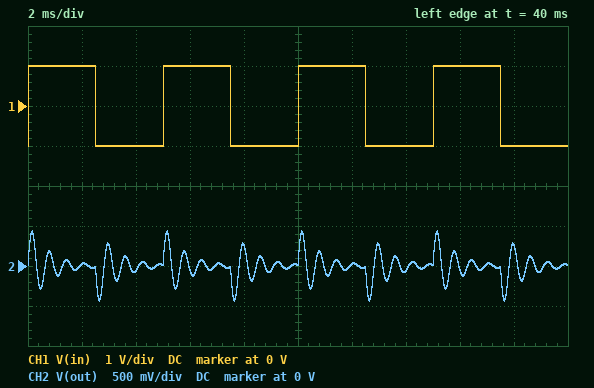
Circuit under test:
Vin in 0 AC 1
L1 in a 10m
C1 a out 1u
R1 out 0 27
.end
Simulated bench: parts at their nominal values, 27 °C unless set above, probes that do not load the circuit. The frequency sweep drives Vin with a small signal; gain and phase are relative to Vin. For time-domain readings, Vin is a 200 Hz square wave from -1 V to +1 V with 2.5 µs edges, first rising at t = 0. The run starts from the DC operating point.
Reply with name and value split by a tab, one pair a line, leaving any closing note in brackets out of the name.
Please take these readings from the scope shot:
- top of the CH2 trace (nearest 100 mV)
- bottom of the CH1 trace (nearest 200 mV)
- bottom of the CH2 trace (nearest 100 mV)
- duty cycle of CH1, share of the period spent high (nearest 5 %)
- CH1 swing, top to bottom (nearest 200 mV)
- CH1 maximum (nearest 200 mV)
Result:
top of the CH2 trace	400 mV
bottom of the CH1 trace	-1.0 V
bottom of the CH2 trace	-400 mV
duty cycle of CH1, share of the period spent high	50 %
CH1 swing, top to bottom	2.0 V
CH1 maximum	1.0 V
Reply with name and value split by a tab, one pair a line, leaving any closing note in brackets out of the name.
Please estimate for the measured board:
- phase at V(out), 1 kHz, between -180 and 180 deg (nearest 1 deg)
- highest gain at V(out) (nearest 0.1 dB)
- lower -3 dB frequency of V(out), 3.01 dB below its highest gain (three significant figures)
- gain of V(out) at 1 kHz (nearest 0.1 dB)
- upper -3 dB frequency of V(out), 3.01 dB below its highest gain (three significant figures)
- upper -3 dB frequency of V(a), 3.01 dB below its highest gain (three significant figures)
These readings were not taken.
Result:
phase at V(out), 1 kHz, between -180 and 180 deg	74 deg
highest gain at V(out)	0 dB
lower -3 dB frequency of V(out), 3.01 dB below its highest gain	1.39 kHz
gain of V(out) at 1 kHz	-11.4 dB
upper -3 dB frequency of V(out), 3.01 dB below its highest gain	1.82 kHz
upper -3 dB frequency of V(a), 3.01 dB below its highest gain	1.77 kHz
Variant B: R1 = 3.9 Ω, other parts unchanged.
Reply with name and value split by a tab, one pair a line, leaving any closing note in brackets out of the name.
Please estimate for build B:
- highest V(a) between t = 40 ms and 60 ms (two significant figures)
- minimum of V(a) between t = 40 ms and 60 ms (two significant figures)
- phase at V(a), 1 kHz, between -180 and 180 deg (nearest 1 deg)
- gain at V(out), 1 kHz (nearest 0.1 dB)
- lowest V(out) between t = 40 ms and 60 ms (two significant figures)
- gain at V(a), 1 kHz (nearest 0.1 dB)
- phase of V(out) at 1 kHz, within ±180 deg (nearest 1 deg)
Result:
highest V(a) between t = 40 ms and 60 ms	2.2 V
minimum of V(a) between t = 40 ms and 60 ms	-2.2 V
phase at V(a), 1 kHz, between -180 and 180 deg	-1 deg
gain at V(out), 1 kHz	-27.9 dB
lowest V(out) between t = 40 ms and 60 ms	-47 mV
gain at V(a), 1 kHz	4.4 dB
phase of V(out) at 1 kHz, within ±180 deg	88 deg
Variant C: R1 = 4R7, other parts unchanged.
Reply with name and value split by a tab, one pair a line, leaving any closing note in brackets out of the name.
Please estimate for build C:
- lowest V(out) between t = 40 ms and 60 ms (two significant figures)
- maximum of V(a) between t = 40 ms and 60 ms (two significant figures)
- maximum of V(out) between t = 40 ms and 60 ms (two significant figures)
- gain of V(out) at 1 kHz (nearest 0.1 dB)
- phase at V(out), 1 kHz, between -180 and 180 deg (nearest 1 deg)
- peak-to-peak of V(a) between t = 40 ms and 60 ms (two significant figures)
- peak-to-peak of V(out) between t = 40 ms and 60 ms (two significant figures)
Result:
lowest V(out) between t = 40 ms and 60 ms	-59 mV
maximum of V(a) between t = 40 ms and 60 ms	2.2 V
maximum of V(out) between t = 40 ms and 60 ms	59 mV
gain of V(out) at 1 kHz	-26.2 dB
phase at V(out), 1 kHz, between -180 and 180 deg	87 deg
peak-to-peak of V(a) between t = 40 ms and 60 ms	4.4 V
peak-to-peak of V(out) between t = 40 ms and 60 ms	120 mV
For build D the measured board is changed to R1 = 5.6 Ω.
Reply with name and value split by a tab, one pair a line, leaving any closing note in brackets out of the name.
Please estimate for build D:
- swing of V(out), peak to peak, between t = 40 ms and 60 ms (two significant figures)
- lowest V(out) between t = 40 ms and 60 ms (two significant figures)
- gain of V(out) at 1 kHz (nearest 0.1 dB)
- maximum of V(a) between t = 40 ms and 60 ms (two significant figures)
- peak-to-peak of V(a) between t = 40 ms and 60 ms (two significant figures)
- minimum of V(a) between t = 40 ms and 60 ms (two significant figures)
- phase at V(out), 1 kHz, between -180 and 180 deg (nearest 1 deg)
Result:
swing of V(out), peak to peak, between t = 40 ms and 60 ms	140 mV
lowest V(out) between t = 40 ms and 60 ms	-72 mV
gain of V(out) at 1 kHz	-24.7 dB
maximum of V(a) between t = 40 ms and 60 ms	2.2 V
peak-to-peak of V(a) between t = 40 ms and 60 ms	4.5 V
minimum of V(a) between t = 40 ms and 60 ms	-2.2 V
phase at V(out), 1 kHz, between -180 and 180 deg	87 deg
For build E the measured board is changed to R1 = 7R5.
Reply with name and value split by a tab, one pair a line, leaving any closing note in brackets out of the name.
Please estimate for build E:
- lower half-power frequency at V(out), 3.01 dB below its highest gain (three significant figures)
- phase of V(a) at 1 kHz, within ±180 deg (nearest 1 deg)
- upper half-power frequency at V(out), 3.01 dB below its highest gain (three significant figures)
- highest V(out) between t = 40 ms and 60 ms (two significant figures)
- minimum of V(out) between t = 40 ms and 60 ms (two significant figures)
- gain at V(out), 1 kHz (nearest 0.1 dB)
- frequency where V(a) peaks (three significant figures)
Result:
lower half-power frequency at V(out), 3.01 dB below its highest gain	1.53 kHz
phase of V(a) at 1 kHz, within ±180 deg	-2 deg
upper half-power frequency at V(out), 3.01 dB below its highest gain	1.65 kHz
highest V(out) between t = 40 ms and 60 ms	100 mV
minimum of V(out) between t = 40 ms and 60 ms	-100 mV
gain at V(out), 1 kHz	-22.2 dB
frequency where V(a) peaks	1.59 kHz
